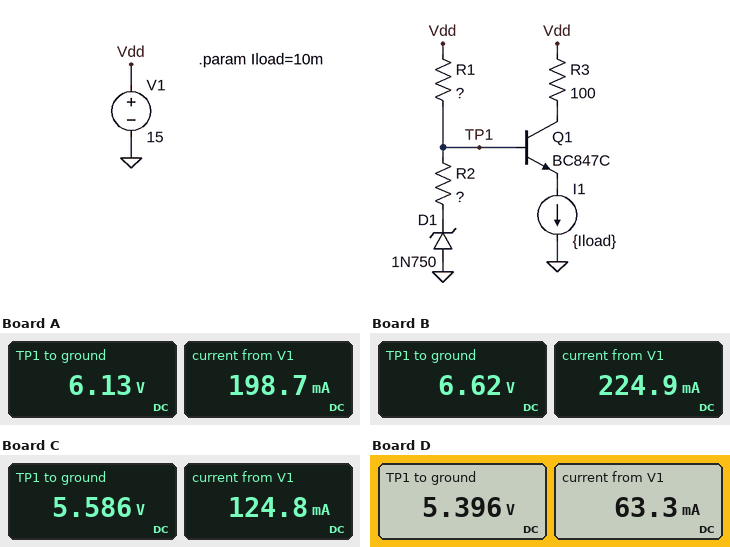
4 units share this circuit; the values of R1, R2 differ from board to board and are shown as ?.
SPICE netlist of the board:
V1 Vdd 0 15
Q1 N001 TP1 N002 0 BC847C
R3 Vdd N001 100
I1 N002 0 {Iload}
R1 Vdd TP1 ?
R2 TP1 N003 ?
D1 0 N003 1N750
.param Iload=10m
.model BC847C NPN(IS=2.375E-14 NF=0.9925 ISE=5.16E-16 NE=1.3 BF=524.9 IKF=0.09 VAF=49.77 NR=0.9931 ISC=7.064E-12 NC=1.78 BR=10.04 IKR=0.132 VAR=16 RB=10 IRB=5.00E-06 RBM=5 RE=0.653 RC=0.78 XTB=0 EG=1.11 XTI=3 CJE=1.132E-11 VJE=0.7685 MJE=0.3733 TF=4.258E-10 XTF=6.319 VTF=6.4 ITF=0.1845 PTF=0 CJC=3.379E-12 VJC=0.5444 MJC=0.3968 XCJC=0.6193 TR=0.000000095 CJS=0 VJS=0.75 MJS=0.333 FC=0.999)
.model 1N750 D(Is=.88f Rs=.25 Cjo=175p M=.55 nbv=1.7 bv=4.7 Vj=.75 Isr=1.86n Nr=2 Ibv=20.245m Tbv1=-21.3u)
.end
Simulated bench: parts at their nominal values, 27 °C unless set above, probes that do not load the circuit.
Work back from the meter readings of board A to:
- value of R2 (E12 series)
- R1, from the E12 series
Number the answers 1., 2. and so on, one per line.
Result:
1. 6.8 Ω
2. 47 Ω
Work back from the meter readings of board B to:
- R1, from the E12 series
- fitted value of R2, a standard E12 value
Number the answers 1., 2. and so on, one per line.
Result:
1. 39 Ω
2. 8.2 Ω
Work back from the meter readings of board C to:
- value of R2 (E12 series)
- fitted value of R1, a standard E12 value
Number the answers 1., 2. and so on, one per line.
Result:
1. 6.8 Ω
2. 82 Ω
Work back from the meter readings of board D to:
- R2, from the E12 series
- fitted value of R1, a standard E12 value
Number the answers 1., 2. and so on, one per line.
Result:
1. 12 Ω
2. 180 Ω
